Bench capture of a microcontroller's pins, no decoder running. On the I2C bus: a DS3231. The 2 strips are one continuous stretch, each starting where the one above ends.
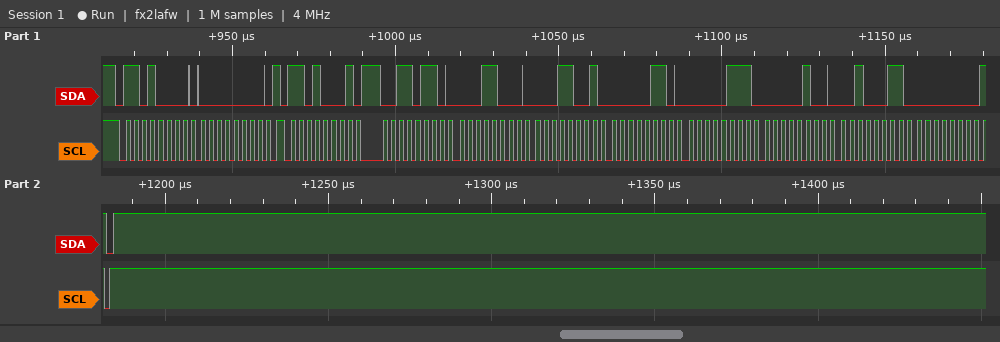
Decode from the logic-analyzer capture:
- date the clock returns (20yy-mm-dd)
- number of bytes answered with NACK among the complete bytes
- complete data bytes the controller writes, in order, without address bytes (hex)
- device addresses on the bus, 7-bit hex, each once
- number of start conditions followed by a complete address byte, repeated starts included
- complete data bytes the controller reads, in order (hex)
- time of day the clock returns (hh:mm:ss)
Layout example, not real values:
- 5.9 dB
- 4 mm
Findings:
- 2023-04-07
- 1
- 00
- 0x68
- 2
- 36 18 19 06 07 04 23 00
- 19:18:36
